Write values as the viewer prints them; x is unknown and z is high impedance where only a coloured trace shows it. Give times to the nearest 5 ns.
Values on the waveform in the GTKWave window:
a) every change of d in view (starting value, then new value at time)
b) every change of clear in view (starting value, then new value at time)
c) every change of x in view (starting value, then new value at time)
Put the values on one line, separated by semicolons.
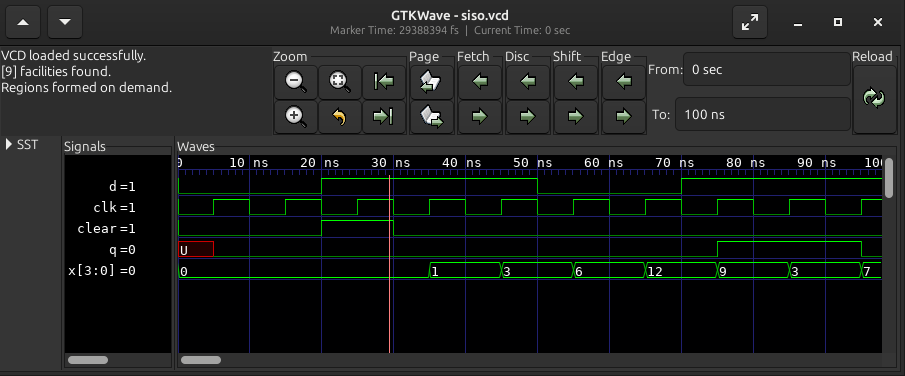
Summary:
0, 1 at 20 ns, 0 at 50 ns, 1 at 70 ns; 0, 1 at 20 ns, 0 at 30 ns; 0, 1 at 35 ns, 3 at 45 ns, 6 at 55 ns, 12 at 65 ns, 9 at 75 ns, 3 at 85 ns, 7 at 95 ns
